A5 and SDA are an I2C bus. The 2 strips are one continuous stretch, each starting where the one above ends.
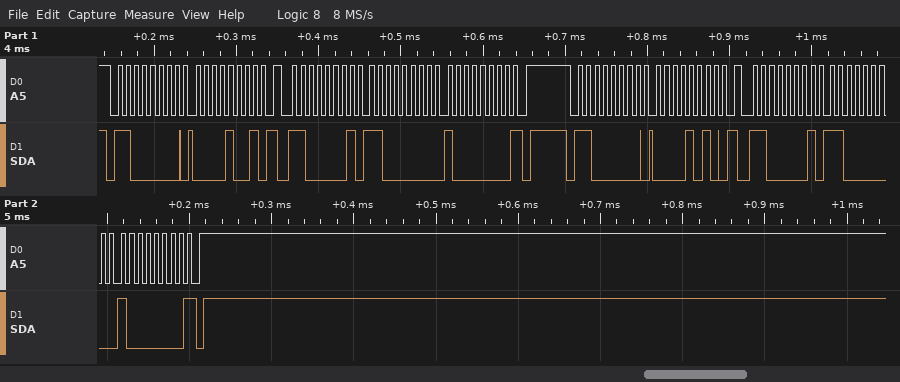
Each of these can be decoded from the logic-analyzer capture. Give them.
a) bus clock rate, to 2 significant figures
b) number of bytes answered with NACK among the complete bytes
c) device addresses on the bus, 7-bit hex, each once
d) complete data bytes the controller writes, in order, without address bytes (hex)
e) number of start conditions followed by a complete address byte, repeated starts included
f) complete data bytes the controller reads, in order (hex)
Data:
100 kHz
2
0x60
09 0A
4
C0 80 C0 80
